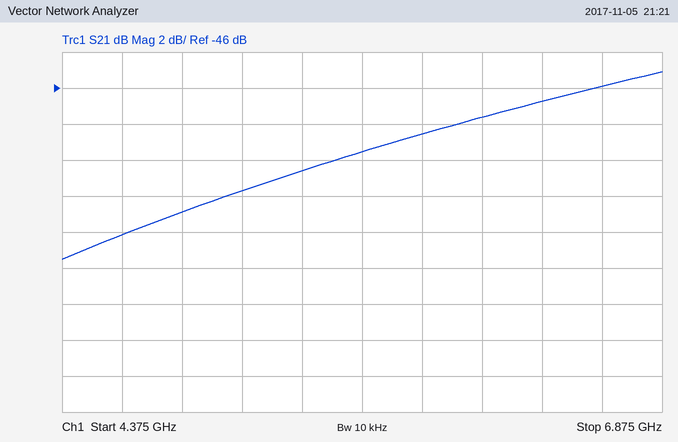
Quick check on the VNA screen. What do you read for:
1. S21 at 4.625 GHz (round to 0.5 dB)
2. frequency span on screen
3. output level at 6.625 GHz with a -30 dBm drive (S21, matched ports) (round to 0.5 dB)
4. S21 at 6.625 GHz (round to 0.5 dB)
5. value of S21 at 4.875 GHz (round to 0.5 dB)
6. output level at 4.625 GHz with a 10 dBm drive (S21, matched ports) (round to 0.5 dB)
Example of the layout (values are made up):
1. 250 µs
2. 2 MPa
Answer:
1. -54.0 dB
2. 2.5 GHz
3. -76.0 dBm
4. -46.0 dB
5. -53.0 dB
6. -44.0 dBm
